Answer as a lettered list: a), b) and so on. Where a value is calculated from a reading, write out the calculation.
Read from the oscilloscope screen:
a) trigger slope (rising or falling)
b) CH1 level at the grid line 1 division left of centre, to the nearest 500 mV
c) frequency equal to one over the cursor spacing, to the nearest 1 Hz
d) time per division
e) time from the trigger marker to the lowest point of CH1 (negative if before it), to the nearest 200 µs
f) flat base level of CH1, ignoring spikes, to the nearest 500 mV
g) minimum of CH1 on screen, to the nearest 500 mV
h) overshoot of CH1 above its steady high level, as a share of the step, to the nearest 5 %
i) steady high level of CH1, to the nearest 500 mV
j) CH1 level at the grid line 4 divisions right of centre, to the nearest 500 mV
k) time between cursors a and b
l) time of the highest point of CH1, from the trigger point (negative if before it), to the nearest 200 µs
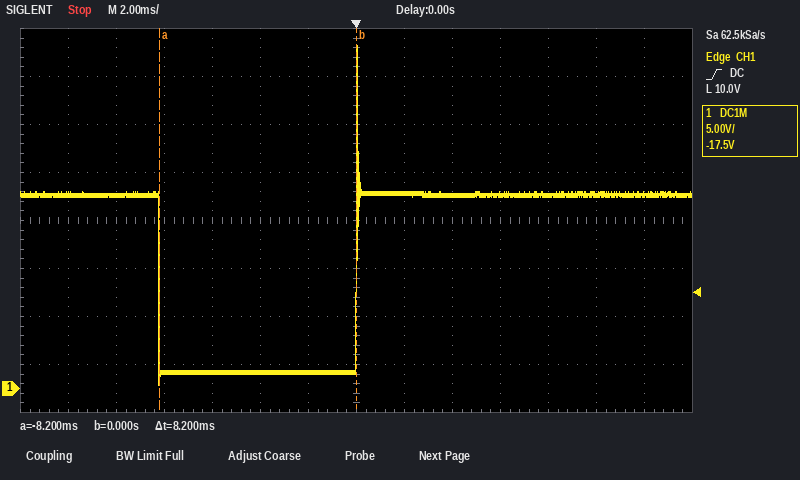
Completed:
a) rising
b) 1.5 V
c) 1 / 8.2 ms ≈ 122 Hz
d) 2 ms
e) -8.2 ms
f) 1.5 V
g) 500 mV
h) 85 %
i) 20.0 V
j) 20.0 V
k) 8.2 ms
l) 0.0 ms
